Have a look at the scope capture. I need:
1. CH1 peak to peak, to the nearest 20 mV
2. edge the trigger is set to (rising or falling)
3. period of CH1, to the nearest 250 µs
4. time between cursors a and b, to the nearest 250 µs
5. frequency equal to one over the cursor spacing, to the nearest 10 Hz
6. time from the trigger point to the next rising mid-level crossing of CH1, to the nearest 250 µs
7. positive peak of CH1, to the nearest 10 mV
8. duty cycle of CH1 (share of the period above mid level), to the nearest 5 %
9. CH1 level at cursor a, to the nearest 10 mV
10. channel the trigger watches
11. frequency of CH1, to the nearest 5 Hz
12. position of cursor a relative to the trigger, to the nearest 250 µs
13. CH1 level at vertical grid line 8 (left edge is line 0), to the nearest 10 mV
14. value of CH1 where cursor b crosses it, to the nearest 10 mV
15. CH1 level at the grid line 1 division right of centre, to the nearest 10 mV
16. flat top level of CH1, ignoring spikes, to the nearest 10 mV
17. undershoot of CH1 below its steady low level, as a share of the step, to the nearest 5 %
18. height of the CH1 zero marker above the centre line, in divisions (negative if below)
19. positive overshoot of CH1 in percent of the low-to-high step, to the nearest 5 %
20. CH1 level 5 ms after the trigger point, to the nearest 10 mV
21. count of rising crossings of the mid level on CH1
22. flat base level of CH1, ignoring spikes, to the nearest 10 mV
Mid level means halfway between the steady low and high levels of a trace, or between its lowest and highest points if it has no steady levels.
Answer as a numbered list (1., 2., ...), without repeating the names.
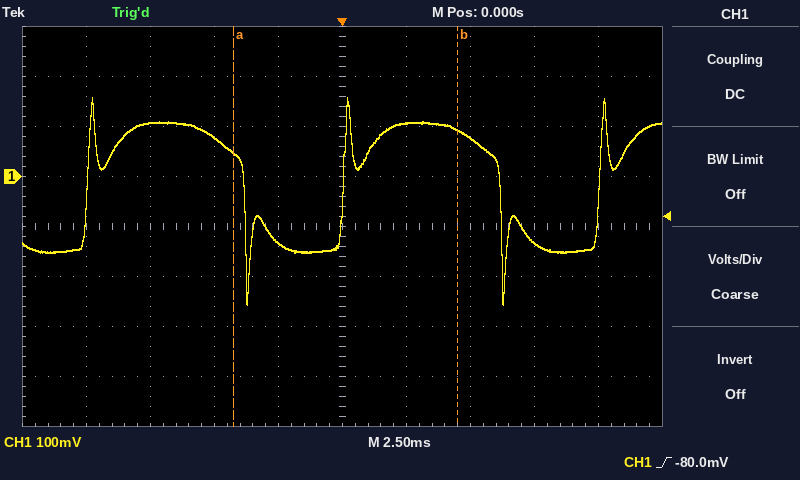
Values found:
1. 420 mV
2. rising
3. 10.00 ms
4. 8.75 ms
5. 110 Hz
6. 10.00 ms
7. 160 mV
8. 60 %
9. 50 mV
10. CH1
11. 100 Hz
12. -4.25 ms
13. -130 mV
14. 90 mV
15. 110 mV
16. 110 mV
17. 40 %
18. +1.0 div
19. 20 %
20. 80 mV
21. 3
22. -150 mV
